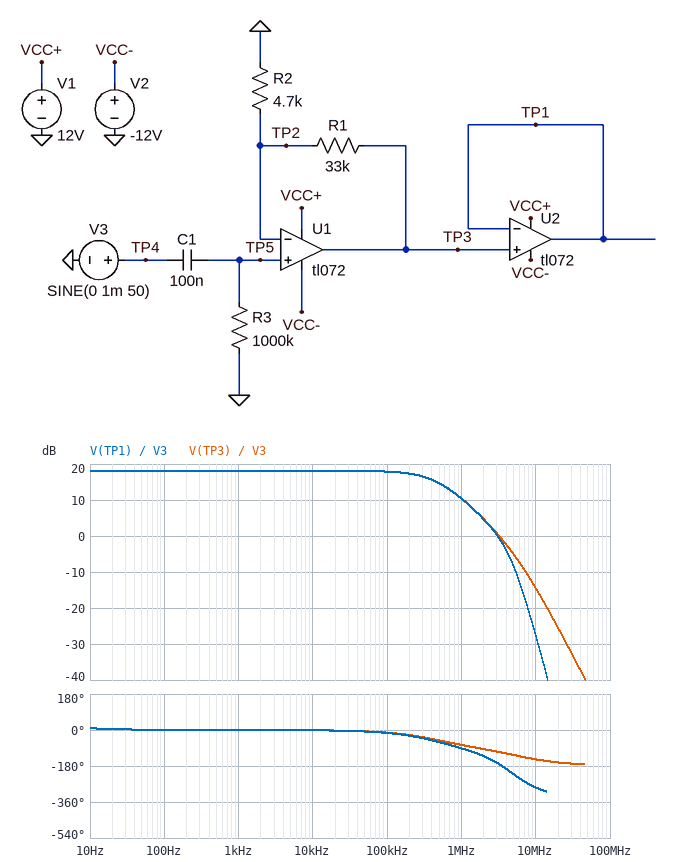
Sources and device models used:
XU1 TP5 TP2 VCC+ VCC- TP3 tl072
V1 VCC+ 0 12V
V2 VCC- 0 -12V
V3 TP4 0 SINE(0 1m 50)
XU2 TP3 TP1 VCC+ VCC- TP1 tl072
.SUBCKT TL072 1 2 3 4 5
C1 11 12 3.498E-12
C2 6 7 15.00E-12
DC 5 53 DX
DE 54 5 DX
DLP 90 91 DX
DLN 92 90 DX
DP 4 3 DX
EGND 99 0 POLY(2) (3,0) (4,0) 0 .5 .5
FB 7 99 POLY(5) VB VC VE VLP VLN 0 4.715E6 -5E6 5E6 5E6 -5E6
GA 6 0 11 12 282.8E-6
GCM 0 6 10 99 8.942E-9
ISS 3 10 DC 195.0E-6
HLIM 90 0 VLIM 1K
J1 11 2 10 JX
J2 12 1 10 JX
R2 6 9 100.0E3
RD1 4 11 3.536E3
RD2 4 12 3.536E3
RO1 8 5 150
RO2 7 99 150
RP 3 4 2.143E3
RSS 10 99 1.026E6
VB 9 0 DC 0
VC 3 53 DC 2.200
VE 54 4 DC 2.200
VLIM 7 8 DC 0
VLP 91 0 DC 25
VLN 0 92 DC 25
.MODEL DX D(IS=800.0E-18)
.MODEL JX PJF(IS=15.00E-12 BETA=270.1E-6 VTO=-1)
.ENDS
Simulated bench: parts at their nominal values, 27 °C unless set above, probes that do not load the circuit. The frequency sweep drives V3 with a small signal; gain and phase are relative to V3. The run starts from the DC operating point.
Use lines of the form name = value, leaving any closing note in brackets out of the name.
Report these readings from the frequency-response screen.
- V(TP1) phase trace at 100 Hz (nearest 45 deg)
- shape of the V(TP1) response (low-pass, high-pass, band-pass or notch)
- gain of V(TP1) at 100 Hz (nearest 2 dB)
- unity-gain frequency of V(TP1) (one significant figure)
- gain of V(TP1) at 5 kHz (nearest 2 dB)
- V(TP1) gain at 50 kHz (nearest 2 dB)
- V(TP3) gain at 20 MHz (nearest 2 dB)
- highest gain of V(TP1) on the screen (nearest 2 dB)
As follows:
V(TP1) phase trace at 100 Hz = 0 deg
shape of the V(TP1) response = low-pass
gain of V(TP1) at 100 Hz = 18 dB
unity-gain frequency of V(TP1) = 3 MHz
gain of V(TP1) at 5 kHz = 18 dB
V(TP1) gain at 50 kHz = 18 dB
V(TP3) gain at 20 MHz = -26 dB
highest gain of V(TP1) on the screen = 18 dB
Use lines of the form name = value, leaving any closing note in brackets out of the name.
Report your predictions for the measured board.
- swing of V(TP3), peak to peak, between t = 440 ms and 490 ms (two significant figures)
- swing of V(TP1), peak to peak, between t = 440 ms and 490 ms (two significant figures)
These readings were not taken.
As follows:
swing of V(TP3), peak to peak, between t = 440 ms and 490 ms = 16 mV
swing of V(TP1), peak to peak, between t = 440 ms and 490 ms = 16 mV
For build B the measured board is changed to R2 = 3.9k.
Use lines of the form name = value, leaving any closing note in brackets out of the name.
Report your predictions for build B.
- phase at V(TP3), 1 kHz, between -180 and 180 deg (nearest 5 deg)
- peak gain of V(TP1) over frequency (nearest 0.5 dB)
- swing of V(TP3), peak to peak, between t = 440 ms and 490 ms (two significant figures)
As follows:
phase at V(TP3), 1 kHz, between -180 and 180 deg = 0 deg
peak gain of V(TP1) over frequency = 19.5 dB
swing of V(TP3), peak to peak, between t = 440 ms and 490 ms = 19 mV
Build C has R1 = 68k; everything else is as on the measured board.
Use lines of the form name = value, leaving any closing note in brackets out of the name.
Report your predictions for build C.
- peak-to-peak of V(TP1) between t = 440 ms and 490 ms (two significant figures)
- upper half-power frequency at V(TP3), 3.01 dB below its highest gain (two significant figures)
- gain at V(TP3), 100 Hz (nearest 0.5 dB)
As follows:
peak-to-peak of V(TP1) between t = 440 ms and 490 ms = 31 mV
upper half-power frequency at V(TP3), 3.01 dB below its highest gain = 230 kHz
gain at V(TP3), 100 Hz = 24.0 dB
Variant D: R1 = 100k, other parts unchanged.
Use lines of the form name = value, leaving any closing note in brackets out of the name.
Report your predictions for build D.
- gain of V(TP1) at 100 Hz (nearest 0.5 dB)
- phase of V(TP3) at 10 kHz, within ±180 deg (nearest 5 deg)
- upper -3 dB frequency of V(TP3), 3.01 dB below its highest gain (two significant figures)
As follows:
gain of V(TP1) at 100 Hz = 27.0 dB
phase of V(TP3) at 10 kHz, within ±180 deg = -5 deg
upper -3 dB frequency of V(TP3), 3.01 dB below its highest gain = 160 kHz
